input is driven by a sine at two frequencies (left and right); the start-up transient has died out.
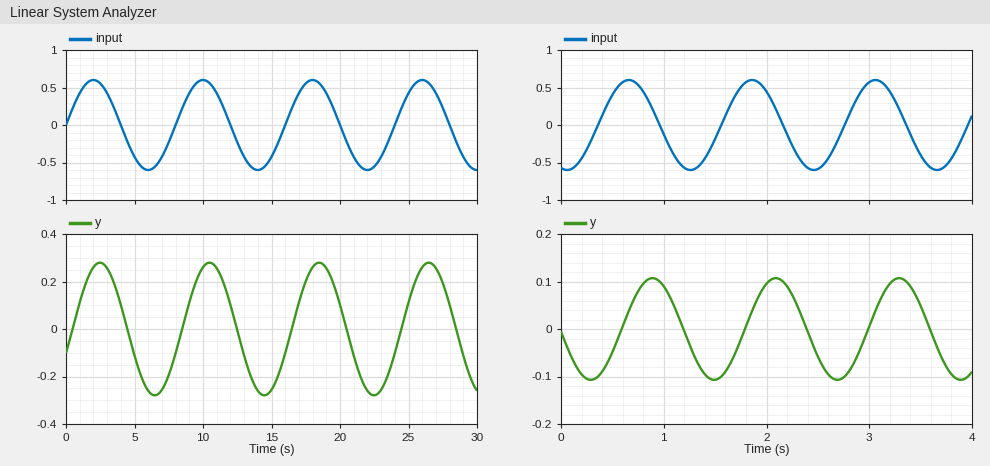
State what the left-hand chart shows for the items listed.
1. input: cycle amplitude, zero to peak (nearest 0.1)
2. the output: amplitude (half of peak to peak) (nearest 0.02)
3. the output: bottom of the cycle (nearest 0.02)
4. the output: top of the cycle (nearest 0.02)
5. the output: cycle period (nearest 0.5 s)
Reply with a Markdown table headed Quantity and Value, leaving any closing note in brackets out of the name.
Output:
| Quantity | Value |
|---|---|
| input: cycle amplitude, zero to peak | 0.6 |
| the output: amplitude (half of peak to peak) | 0.28 |
| the output: bottom of the cycle | -0.28 |
| the output: top of the cycle | 0.28 |
| the output: cycle period | 8.0 s |
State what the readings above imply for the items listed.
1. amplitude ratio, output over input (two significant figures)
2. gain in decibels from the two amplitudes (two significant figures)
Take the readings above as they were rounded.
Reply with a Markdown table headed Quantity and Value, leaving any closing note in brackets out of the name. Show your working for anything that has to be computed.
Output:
| Quantity | Value |
|---|---|
| amplitude ratio, output over input | 0.28 / 0.6 = 0.47 |
| gain in decibels from the two amplitudes | 20 log10(0.28 / 0.6) = -6.6 dB |
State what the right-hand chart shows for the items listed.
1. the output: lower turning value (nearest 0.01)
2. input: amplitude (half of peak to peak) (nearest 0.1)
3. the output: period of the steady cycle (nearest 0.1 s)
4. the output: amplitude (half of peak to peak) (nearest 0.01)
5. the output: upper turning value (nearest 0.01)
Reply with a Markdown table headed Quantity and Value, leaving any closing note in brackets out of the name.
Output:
| Quantity | Value |
|---|---|
| the output: lower turning value | -0.11 |
| input: amplitude (half of peak to peak) | 0.6 |
| the output: period of the steady cycle | 1.2 s |
| the output: amplitude (half of peak to peak) | 0.11 |
| the output: upper turning value | 0.11 |
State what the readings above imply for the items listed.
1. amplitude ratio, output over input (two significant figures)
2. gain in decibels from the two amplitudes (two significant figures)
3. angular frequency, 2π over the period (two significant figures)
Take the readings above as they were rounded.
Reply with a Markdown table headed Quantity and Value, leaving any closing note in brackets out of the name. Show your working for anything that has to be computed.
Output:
| Quantity | Value |
|---|---|
| amplitude ratio, output over input | 0.11 / 0.6 = 0.18 |
| gain in decibels from the two amplitudes | 20 log10(0.11 / 0.6) = -15 dB |
| angular frequency, 2π over the period | 2π / 1.2 = 5.2 rad/s |
